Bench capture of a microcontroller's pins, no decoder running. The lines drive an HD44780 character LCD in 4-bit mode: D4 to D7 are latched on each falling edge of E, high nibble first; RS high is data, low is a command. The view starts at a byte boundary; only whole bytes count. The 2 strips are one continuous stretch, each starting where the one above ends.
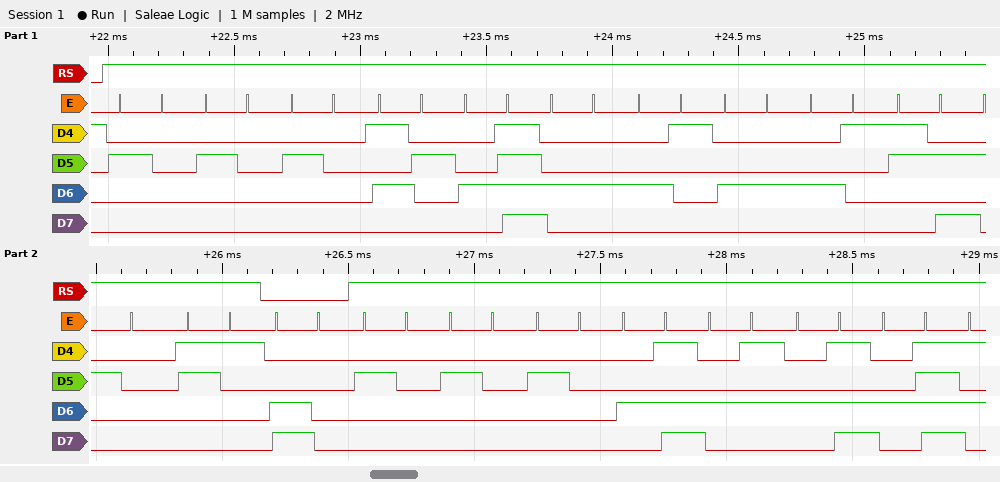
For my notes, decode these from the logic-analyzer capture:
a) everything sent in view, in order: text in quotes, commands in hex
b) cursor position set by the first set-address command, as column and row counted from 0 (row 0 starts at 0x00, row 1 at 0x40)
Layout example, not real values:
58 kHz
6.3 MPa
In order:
"   RODADA: 1" 0xC0 "   MEMO"
column 0, row 1
